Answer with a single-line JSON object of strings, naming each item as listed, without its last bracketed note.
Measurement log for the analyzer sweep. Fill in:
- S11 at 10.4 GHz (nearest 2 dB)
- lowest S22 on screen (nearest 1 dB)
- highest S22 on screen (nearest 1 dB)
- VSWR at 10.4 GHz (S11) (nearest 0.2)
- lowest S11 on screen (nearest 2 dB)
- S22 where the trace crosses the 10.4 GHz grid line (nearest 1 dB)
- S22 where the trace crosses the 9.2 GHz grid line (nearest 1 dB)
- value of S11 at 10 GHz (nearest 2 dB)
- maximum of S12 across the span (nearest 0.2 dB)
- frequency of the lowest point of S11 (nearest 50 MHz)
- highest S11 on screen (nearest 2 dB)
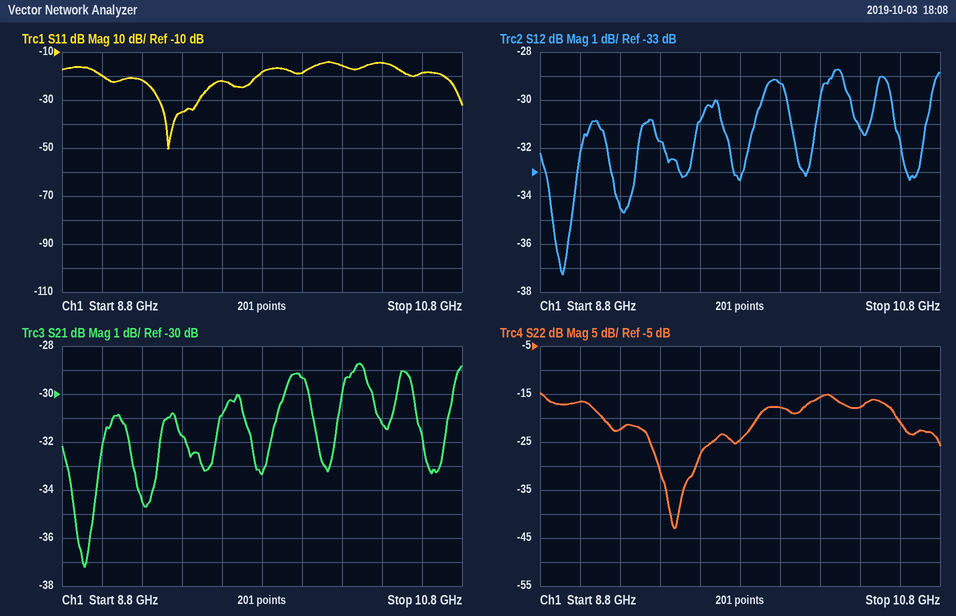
{"S11 at 10.4 GHz": "-14 dB", "lowest S22 on screen": "-43 dB", "highest S22 on screen": "-15 dB", "VSWR at 10.4 GHz (S11)": "1.4", "lowest S11 on screen": "-50 dB", "S22 where the trace crosses the 10.4 GHz grid line": "-18 dB", "S22 where the trace crosses the 9.2 GHz grid line": "-22 dB", "value of S11 at 10 GHz": "-18 dB", "maximum of S12 across the span": "-28.8 dB", "frequency of the lowest point of S11": "9.35 GHz", "highest S11 on screen": "-14 dB"}
